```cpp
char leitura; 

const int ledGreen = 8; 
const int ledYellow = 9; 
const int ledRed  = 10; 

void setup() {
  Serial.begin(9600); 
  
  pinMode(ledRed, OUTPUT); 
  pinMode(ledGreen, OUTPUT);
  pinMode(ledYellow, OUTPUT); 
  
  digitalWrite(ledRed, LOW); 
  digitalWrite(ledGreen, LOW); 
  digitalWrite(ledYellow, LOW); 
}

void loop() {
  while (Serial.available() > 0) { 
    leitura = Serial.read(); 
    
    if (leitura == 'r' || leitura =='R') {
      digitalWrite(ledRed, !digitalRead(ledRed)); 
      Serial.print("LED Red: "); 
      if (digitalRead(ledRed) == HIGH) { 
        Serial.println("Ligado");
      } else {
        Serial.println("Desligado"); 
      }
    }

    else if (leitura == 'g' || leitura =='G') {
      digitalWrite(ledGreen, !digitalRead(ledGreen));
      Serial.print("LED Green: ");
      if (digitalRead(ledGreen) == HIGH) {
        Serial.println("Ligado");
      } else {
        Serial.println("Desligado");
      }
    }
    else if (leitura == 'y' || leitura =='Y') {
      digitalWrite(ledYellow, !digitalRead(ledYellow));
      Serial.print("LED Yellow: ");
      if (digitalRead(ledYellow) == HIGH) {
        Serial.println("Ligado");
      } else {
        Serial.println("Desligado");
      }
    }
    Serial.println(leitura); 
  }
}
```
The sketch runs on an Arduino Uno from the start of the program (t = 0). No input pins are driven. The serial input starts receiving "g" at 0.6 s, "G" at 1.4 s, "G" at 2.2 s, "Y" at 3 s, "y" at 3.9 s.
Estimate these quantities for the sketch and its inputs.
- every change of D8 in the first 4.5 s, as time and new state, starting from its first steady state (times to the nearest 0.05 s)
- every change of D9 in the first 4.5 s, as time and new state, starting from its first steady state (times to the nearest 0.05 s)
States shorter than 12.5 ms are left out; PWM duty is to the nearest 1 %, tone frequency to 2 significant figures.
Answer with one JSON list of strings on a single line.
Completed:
["0 s low; 0.6 s high; 1.4 s low; 2.2 s high", "0 s low; 3 s high; 3.9 s low"]
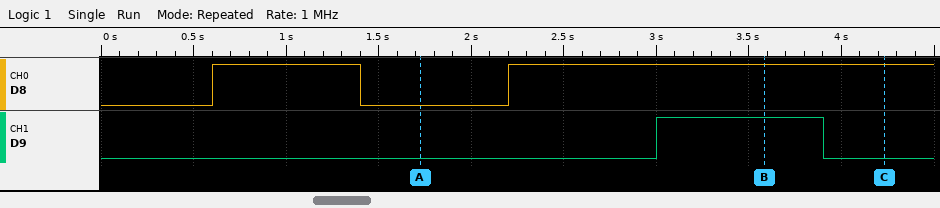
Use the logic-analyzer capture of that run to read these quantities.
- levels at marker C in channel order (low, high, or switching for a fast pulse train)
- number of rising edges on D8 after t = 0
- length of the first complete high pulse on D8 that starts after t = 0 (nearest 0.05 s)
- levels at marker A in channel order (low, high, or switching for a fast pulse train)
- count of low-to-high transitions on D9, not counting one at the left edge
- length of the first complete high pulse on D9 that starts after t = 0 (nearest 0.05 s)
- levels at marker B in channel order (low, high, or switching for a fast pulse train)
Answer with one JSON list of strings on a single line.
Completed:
["D8 high, D9 low", "2", "0.80 s", "D8 low, D9 low", "1", "0.90 s", "D8 high, D9 high"]
